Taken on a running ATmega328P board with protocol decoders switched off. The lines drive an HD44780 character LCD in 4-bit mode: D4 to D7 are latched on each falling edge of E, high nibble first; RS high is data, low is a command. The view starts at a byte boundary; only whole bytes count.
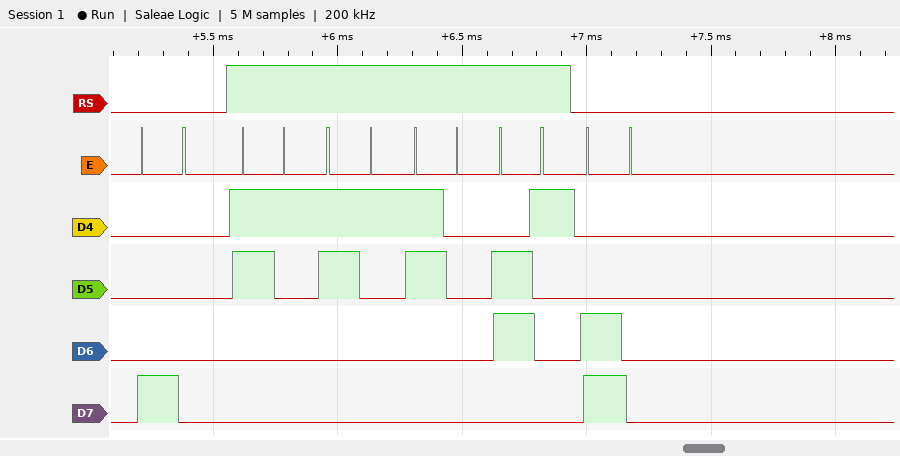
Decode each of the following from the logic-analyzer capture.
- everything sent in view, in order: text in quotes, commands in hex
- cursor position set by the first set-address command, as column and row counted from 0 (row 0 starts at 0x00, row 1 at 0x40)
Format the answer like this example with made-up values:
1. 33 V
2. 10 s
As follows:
1. 0x80 "110a" 0xC0
2. column 0, row 0
